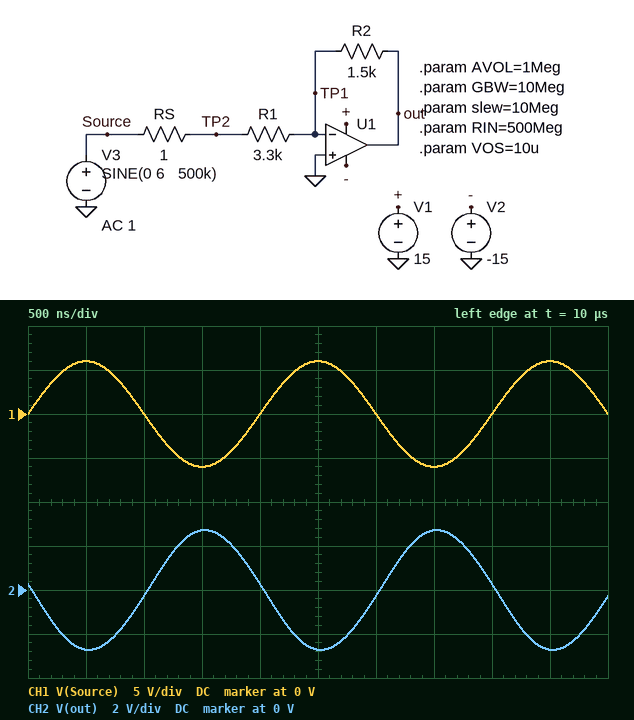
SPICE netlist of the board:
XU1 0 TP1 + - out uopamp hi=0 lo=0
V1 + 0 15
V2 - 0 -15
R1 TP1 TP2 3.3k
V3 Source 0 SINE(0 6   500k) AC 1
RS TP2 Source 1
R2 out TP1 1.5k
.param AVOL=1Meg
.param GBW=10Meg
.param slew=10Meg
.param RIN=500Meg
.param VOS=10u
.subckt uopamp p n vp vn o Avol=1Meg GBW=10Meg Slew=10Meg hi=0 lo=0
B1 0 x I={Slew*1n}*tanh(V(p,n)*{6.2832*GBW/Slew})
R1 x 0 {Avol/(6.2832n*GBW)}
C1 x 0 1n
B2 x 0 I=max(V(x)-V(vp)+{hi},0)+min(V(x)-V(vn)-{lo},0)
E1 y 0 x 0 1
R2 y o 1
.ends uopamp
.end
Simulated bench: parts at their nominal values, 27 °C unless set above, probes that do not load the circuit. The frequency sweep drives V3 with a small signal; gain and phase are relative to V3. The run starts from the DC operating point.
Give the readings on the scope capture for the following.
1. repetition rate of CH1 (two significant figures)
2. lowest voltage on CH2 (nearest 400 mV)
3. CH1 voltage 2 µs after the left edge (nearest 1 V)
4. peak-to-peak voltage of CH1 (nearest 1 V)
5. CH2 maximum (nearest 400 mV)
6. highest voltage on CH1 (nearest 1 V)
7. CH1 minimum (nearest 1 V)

500 kHz
-2.8 V
0 V
12 V
2.8 V
6 V
-6 V
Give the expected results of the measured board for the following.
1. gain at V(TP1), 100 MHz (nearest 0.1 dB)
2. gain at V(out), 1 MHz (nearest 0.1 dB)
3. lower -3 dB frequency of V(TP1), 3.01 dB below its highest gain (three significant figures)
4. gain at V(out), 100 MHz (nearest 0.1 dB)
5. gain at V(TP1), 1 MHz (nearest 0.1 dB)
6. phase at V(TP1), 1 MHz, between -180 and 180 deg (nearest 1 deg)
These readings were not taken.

-10.1 dB
-6.9 dB
6.87 MHz
-30.1 dB
-26.9 dB
82 deg
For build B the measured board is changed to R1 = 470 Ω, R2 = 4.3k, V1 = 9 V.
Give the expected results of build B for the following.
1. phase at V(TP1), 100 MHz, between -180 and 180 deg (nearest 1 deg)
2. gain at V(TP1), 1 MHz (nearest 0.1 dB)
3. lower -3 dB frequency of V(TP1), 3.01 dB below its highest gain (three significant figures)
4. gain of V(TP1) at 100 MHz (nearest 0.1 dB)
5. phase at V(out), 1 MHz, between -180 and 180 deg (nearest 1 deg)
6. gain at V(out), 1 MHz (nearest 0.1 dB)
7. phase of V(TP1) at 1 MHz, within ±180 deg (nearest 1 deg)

1 deg
-3.9 dB
987 kHz
-0.9 dB
135 deg
16.1 dB
45 deg
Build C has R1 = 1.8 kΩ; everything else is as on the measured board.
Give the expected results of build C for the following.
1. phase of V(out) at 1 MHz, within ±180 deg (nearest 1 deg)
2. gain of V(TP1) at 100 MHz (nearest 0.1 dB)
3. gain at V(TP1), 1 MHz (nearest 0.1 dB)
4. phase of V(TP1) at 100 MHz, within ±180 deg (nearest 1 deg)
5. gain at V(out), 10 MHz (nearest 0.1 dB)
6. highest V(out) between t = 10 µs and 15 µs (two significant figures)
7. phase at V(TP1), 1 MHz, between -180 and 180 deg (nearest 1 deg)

170 deg
-6.9 dB
-21.7 dB
3 deg
-8.0 dB
4.6 V
80 deg
